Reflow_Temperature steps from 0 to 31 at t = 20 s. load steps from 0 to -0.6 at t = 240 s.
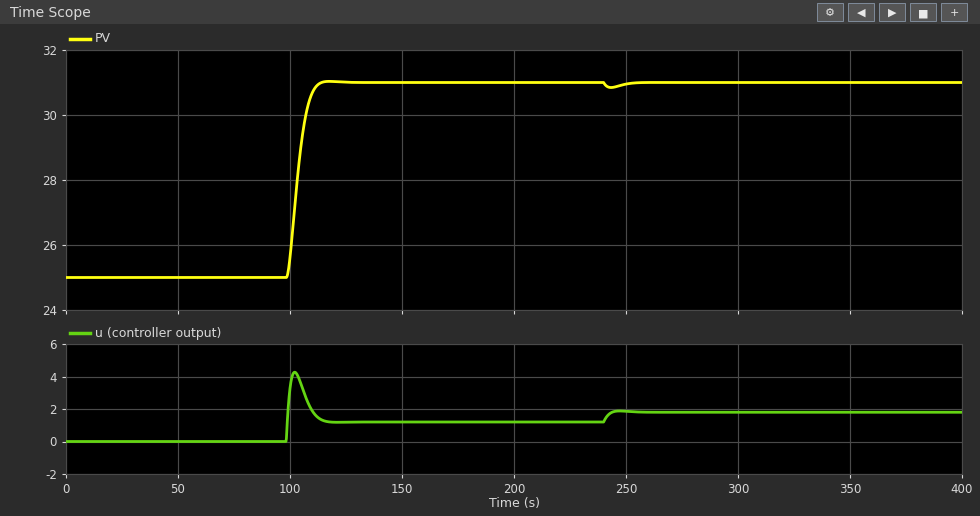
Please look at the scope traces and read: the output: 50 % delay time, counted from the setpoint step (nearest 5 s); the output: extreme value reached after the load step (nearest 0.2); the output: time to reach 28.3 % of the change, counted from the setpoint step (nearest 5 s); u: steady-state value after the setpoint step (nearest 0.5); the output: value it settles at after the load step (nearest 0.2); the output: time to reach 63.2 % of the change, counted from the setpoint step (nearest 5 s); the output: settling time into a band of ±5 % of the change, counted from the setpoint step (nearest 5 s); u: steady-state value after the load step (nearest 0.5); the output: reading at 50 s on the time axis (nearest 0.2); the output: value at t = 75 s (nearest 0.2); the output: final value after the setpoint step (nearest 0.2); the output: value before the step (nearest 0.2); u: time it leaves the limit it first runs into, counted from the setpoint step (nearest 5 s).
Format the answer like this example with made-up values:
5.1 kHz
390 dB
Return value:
85 s
30.8
80 s
1.0
31.0
85 s
90 s
2.0
25.0
25.0
31.0
25.0
80 s
